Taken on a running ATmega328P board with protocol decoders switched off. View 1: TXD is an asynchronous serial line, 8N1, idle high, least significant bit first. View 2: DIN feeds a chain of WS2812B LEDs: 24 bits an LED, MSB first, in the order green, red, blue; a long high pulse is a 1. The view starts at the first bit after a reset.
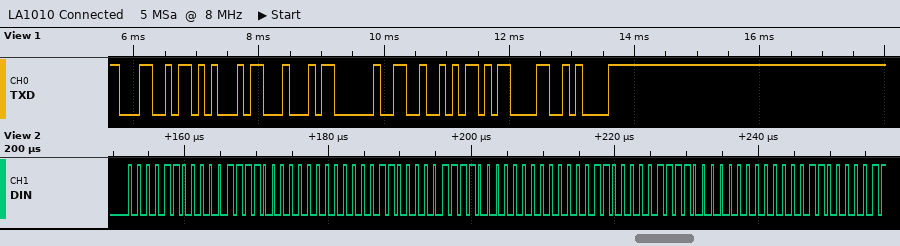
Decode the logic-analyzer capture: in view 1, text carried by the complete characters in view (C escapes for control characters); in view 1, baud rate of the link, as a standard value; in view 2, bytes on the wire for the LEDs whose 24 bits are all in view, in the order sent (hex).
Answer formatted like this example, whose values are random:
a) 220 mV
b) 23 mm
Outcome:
a) "LED R\r\n"
b) 9600 baud
c) 0C 1E 00 0C 1E 00 0C 1E 00
